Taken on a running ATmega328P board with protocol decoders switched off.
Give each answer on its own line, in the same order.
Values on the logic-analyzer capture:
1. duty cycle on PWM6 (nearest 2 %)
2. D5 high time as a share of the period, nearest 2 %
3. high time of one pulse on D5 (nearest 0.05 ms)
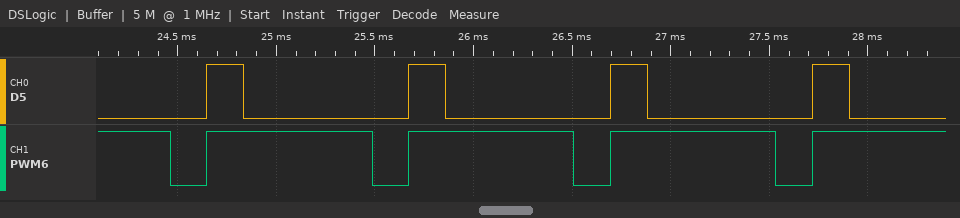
82 %
18 %
0.20 ms
